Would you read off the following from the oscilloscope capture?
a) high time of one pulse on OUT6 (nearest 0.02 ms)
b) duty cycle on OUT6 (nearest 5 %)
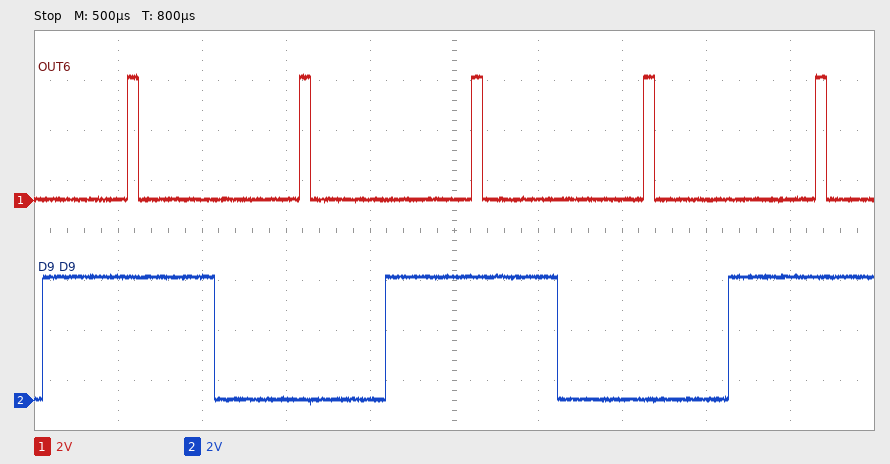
0.06 ms
5 %
